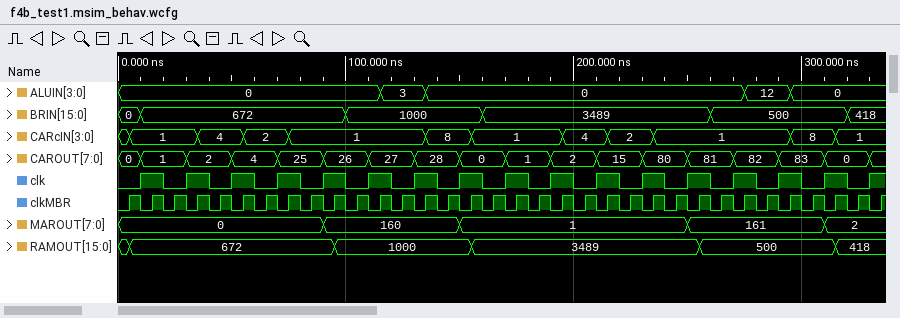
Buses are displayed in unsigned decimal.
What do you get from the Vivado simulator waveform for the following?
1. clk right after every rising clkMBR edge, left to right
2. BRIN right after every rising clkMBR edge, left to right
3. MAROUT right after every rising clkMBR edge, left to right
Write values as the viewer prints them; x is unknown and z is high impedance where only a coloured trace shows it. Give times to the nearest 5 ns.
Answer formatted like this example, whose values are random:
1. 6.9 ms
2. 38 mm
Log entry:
1. 0 1 0 1 0 1 0 1 0 1 0 1 0 1 0 1 0 1 0 1 0 1 0 1 0 1 0 1 0 1 0 1 0 1
2. 0, 672, 672, 672, 672, 672, 672, 672, 672, 672, 1000, 1000, 1000, 1000, 1000, 1000, 3489, 3489, 3489, 3489, 3489, 3489, 3489, 3489, 3489, 3489, 500, 500, 500, 500, 500, 500, 418, 418
3. 0, 0, 0, 0, 0, 0, 0, 0, 0, 160, 160, 160, 160, 160, 160, 1, 1, 1, 1, 1, 1, 1, 1, 1, 1, 161, 161, 161, 161, 161, 161, 2, 2, 2
